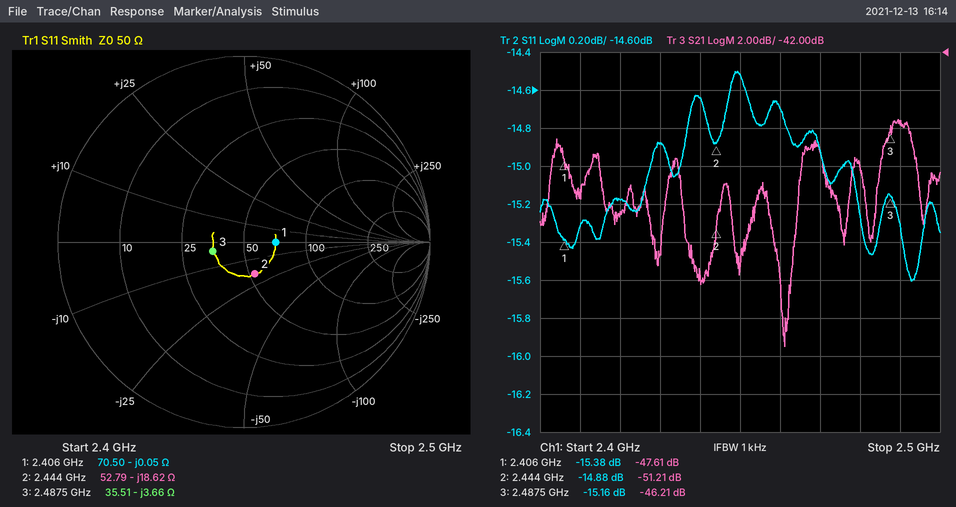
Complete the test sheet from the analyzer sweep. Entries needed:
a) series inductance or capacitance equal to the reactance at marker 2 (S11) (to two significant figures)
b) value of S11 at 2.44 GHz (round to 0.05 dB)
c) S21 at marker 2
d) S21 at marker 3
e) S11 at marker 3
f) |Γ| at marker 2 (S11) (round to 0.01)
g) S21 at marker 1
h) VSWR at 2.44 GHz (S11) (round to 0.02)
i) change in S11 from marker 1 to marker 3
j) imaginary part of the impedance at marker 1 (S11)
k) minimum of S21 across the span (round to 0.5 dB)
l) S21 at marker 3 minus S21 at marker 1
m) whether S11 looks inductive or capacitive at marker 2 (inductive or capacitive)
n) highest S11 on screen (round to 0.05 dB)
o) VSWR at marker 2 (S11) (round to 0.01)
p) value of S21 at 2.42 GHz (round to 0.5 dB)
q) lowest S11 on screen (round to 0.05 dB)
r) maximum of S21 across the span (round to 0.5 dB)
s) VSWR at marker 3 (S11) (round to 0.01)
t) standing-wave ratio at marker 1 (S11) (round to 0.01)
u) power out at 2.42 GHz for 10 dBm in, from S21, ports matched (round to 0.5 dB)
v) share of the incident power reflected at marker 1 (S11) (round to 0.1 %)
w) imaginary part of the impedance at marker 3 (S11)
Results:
3.5 pF
-14.65 dB
-51.21 dB
-46.21 dB
-15.16 dB
0.18
-47.61 dB
1.46
0.22 dB
-0.05 Ω
-57.5 dB
1.40 dB
capacitive
-14.50 dB
1.44
-50.5 dB
-15.60 dB
-45.5 dB
1.42
1.41
-40.5 dBm
2.9 %
-3.66 Ω
